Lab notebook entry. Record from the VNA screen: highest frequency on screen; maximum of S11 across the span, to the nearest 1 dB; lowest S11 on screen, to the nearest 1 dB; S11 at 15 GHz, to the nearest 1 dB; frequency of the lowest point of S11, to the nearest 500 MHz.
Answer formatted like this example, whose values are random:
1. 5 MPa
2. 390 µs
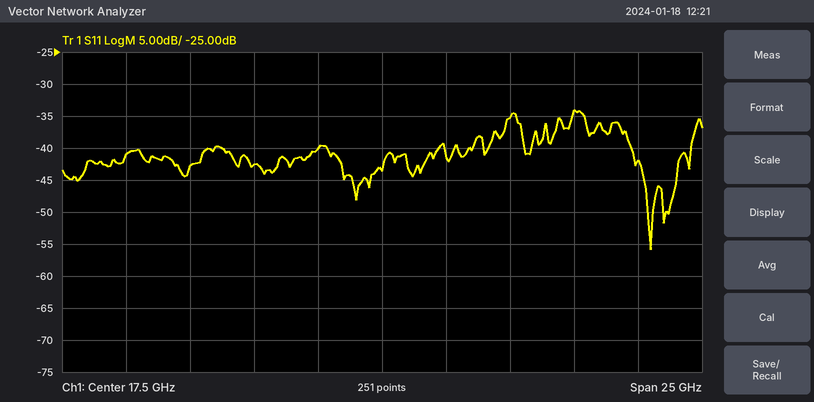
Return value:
1. 30 GHz
2. -34 dB
3. -56 dB
4. -40 dB
5. 28.0 GHz
